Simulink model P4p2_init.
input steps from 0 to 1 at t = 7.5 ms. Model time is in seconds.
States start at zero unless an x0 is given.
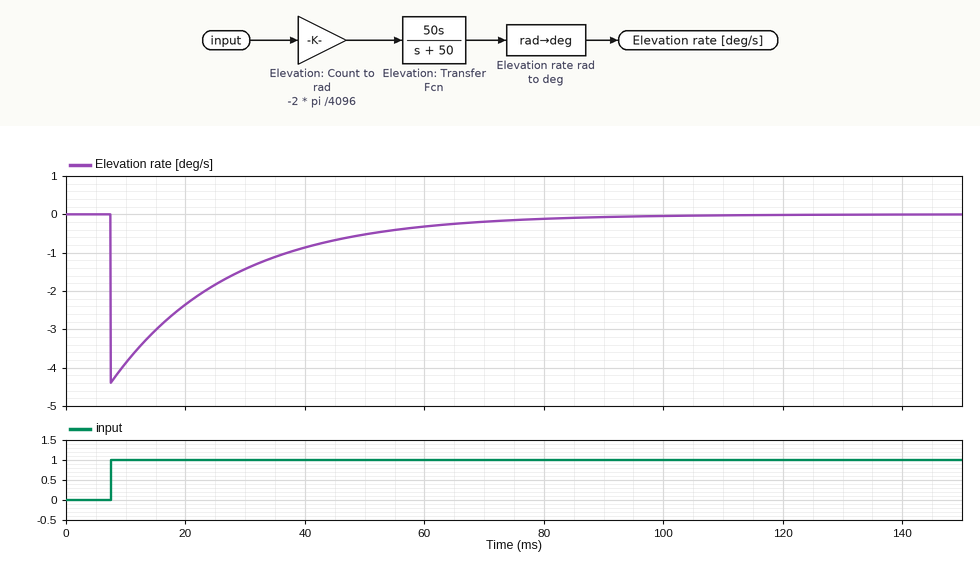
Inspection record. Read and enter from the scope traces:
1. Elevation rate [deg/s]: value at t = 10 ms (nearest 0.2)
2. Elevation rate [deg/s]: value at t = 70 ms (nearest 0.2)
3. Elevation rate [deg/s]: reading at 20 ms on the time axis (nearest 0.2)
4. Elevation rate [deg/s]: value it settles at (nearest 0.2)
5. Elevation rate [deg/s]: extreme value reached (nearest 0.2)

-3.8
-0.2
-2.4
0.0
-4.4
